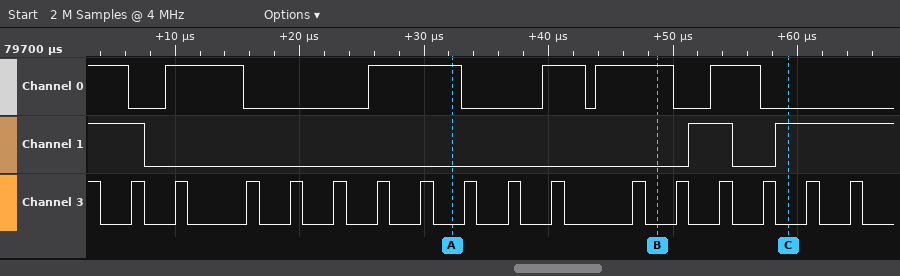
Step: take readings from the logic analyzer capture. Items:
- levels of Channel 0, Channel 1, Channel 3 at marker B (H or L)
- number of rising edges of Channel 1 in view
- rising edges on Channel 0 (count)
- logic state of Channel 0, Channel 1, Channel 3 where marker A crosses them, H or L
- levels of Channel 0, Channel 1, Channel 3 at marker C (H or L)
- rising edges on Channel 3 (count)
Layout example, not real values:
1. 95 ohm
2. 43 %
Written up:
1. Channel 0=H, Channel 1=L, Channel 3=L
2. 2
3. 5
4. Channel 0=H, Channel 1=L, Channel 3=L
5. Channel 0=L, Channel 1=H, Channel 3=L
6. 16
